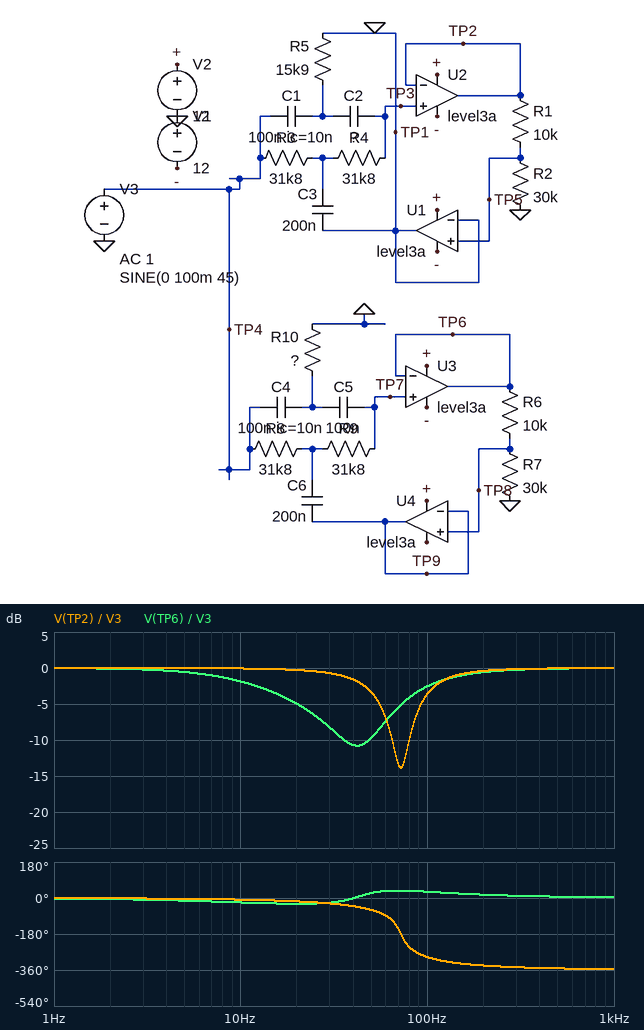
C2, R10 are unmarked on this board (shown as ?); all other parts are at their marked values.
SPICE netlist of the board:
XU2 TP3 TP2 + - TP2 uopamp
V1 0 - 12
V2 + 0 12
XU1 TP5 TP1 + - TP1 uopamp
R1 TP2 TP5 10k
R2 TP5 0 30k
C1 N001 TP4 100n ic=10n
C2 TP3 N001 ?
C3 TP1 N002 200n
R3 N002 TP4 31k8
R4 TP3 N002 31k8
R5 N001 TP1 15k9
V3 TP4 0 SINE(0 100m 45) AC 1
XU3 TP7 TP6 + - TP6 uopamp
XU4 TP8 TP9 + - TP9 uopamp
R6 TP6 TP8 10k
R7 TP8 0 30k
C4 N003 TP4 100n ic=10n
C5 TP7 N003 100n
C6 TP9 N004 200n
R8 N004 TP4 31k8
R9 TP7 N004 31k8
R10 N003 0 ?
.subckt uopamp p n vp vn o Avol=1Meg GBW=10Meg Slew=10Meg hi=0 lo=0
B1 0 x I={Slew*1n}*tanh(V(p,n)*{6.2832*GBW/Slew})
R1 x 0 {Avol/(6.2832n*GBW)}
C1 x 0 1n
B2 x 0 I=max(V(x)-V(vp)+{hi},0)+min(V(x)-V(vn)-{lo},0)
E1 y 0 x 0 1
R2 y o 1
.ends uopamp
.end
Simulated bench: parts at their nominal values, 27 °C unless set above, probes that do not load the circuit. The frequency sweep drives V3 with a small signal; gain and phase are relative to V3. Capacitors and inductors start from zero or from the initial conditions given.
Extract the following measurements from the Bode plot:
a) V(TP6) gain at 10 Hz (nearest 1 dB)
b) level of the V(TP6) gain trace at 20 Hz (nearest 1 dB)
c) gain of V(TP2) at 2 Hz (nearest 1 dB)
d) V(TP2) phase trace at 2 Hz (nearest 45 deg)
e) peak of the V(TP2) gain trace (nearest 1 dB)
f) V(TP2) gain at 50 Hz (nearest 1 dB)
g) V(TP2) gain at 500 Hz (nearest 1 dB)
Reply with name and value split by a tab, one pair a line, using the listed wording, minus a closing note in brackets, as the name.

V(TP6) gain at 10 Hz	-2 dB
level of the V(TP6) gain trace at 20 Hz	-5 dB
gain of V(TP2) at 2 Hz	0 dB
V(TP2) phase trace at 2 Hz	0 deg
peak of the V(TP2) gain trace	0 dB
V(TP2) gain at 50 Hz	-3 dB
V(TP2) gain at 500 Hz	0 dB
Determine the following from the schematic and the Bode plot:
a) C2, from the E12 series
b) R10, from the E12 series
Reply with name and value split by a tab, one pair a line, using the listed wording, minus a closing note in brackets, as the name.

C2, from the E12 series	39 nF
R10, from the E12 series	47 kΩ
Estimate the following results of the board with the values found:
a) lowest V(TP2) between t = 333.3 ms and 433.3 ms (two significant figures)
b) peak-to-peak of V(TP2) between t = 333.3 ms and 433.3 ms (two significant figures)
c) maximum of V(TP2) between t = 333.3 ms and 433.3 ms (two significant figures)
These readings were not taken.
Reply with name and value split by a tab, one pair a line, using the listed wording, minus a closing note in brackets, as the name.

lowest V(TP2) between t = 333.3 ms and 433.3 ms	-77 mV
peak-to-peak of V(TP2) between t = 333.3 ms and 433.3 ms	150 mV
maximum of V(TP2) between t = 333.3 ms and 433.3 ms	77 mV
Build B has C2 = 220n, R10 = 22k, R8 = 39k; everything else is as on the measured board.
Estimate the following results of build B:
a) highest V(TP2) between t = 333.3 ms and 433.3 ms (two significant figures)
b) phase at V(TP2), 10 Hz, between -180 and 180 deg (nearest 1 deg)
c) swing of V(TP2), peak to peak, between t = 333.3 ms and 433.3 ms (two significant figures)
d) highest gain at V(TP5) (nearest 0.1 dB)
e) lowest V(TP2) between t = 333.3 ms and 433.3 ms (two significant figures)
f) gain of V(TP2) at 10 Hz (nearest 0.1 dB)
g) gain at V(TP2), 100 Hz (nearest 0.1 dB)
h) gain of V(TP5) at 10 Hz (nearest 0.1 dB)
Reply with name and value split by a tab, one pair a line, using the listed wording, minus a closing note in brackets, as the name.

highest V(TP2) between t = 333.3 ms and 433.3 ms	30 mV
phase at V(TP2), 10 Hz, between -180 and 180 deg	-18 deg
swing of V(TP2), peak to peak, between t = 333.3 ms and 433.3 ms	60 mV
highest gain at V(TP5)	-2.5 dB
lowest V(TP2) between t = 333.3 ms and 433.3 ms	-30 mV
gain of V(TP2) at 10 Hz	-0.7 dB
gain at V(TP2), 100 Hz	-1.3 dB
gain of V(TP5) at 10 Hz	-3.2 dB
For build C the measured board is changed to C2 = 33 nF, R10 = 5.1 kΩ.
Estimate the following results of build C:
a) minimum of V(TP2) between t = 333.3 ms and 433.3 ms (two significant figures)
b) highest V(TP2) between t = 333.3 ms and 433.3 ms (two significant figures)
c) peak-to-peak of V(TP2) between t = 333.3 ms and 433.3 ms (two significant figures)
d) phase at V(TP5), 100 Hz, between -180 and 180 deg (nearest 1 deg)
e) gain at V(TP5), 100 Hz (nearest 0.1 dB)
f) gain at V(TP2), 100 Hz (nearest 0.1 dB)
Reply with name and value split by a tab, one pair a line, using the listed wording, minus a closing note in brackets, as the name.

minimum of V(TP2) between t = 333.3 ms and 433.3 ms	-81 mV
highest V(TP2) between t = 333.3 ms and 433.3 ms	81 mV
peak-to-peak of V(TP2) between t = 333.3 ms and 433.3 ms	160 mV
phase at V(TP5), 100 Hz, between -180 and 180 deg	77 deg
gain at V(TP5), 100 Hz	-7.2 dB
gain at V(TP2), 100 Hz	-4.7 dB
